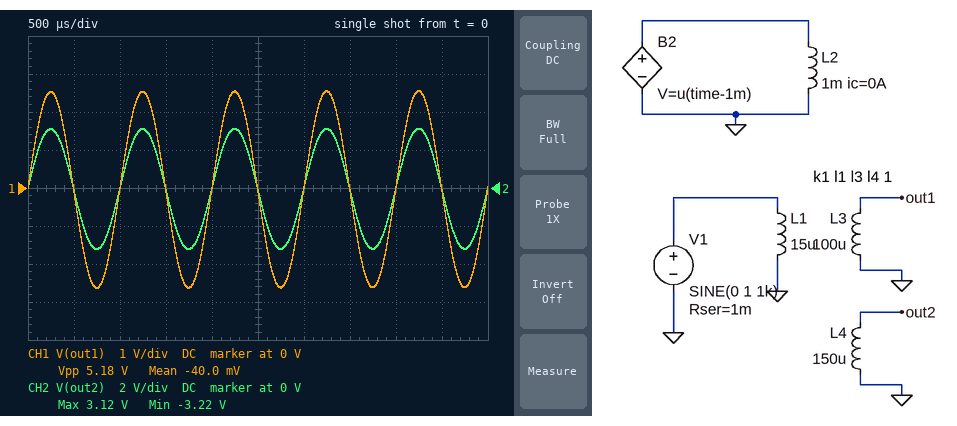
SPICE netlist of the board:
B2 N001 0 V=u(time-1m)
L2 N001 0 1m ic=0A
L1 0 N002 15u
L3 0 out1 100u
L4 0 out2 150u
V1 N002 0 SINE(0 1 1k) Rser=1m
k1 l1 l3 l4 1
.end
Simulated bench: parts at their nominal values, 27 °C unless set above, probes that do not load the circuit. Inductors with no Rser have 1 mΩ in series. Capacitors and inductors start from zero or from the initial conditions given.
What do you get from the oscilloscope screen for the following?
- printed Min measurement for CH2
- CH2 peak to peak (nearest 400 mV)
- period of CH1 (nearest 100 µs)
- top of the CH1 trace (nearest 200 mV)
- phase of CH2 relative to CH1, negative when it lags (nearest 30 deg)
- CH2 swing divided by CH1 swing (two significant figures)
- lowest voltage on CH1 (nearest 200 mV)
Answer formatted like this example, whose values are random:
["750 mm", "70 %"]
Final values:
["-3.22 V", "6.4 V", "1.0 ms", "2.6 V", "0 deg", "1.2", "-2.6 V"]
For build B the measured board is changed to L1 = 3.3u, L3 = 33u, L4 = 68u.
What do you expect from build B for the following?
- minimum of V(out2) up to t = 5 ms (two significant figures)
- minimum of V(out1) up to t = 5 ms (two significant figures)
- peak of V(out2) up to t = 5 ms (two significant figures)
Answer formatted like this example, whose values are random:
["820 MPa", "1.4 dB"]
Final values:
["-4.8 V", "-3.3 V", "4.5 V"]
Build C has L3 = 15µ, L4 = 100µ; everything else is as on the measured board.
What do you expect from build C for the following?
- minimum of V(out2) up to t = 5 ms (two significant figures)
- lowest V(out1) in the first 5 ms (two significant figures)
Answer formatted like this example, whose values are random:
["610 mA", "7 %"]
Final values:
["-2.6 V", "-1.0 V"]
